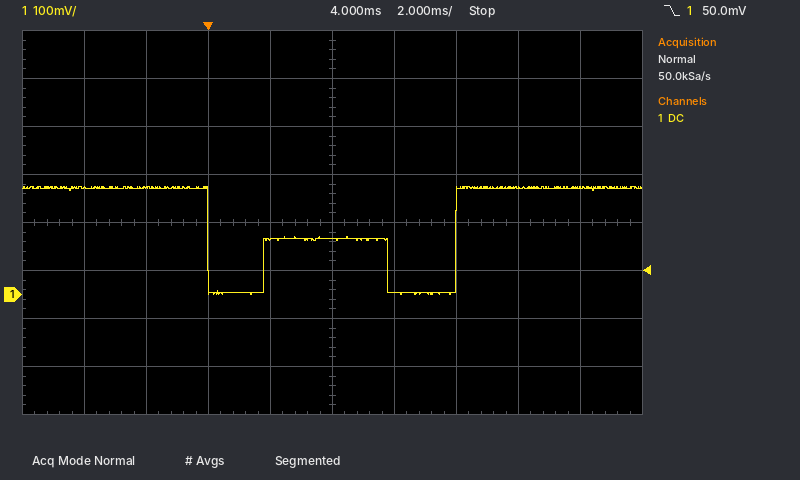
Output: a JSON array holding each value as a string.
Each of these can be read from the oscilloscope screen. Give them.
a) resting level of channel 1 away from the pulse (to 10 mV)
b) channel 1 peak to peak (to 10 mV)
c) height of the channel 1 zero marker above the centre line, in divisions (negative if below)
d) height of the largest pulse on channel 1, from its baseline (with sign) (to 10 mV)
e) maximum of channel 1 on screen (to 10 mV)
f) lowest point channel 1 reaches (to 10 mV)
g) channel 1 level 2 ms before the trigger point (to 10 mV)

["220 mV", "220 mV", "-1.5 div", "-220 mV", "220 mV", "0 mV", "220 mV"]
